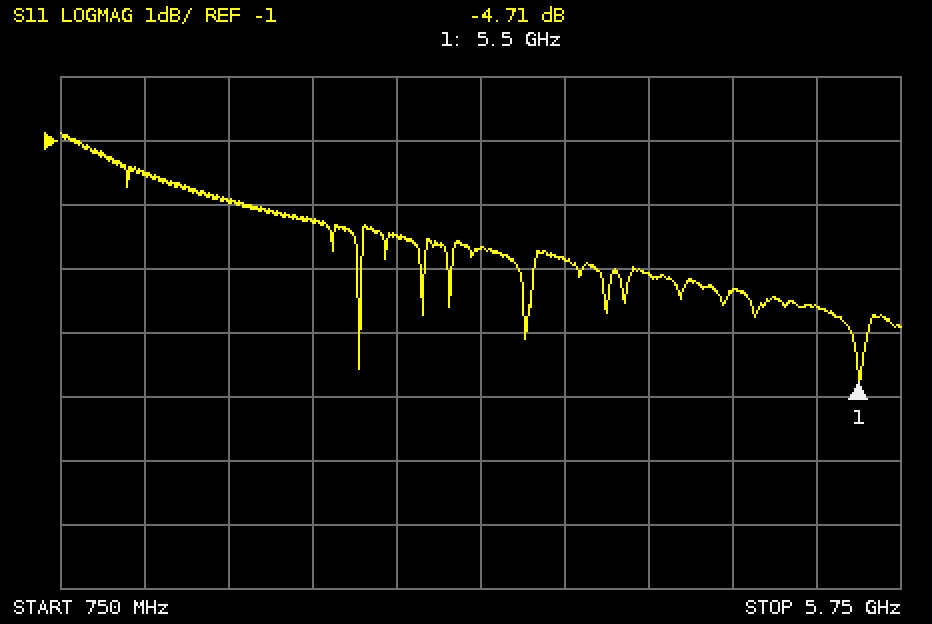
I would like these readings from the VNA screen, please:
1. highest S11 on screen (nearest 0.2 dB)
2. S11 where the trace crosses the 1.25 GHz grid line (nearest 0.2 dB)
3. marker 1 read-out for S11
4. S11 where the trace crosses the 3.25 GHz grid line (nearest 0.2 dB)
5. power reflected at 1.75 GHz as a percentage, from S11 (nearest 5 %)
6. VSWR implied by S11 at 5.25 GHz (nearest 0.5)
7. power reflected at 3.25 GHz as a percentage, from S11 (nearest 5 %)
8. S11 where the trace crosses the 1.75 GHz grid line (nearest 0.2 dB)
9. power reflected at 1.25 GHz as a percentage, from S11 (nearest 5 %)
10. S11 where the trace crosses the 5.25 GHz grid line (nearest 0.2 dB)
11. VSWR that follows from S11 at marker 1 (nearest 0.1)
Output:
-0.8 dB
-1.6 dB
-4.71 dB
-2.6 dB
65 %
5.0
55 %
-2.0 dB
70 %
-3.6 dB
3.8
